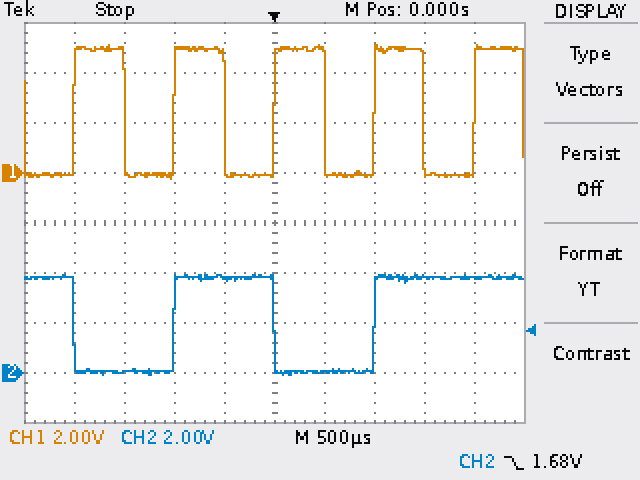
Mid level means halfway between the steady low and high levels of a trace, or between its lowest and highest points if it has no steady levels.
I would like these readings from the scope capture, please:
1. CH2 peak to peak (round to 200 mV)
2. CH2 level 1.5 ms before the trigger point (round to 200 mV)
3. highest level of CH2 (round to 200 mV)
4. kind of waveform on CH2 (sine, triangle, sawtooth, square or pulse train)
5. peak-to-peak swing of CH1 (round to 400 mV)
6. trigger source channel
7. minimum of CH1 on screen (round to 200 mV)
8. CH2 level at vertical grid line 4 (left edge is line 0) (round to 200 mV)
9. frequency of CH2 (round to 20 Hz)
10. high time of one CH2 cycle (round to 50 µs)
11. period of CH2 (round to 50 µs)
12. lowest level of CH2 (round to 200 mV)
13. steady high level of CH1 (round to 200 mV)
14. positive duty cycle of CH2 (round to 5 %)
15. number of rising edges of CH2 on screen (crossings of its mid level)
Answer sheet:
4.0 V
0.0 V
4.0 V
square
5.2 V
CH2
-200 mV
3.8 V
500 Hz
1.00 ms
2.00 ms
0.0 V
5.0 V
50 %
2
